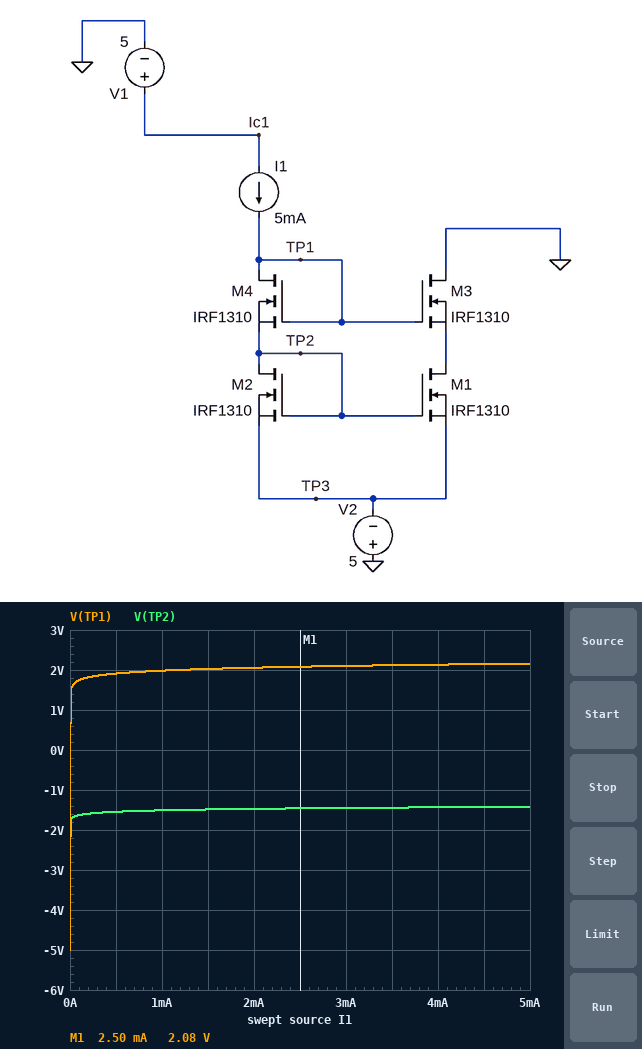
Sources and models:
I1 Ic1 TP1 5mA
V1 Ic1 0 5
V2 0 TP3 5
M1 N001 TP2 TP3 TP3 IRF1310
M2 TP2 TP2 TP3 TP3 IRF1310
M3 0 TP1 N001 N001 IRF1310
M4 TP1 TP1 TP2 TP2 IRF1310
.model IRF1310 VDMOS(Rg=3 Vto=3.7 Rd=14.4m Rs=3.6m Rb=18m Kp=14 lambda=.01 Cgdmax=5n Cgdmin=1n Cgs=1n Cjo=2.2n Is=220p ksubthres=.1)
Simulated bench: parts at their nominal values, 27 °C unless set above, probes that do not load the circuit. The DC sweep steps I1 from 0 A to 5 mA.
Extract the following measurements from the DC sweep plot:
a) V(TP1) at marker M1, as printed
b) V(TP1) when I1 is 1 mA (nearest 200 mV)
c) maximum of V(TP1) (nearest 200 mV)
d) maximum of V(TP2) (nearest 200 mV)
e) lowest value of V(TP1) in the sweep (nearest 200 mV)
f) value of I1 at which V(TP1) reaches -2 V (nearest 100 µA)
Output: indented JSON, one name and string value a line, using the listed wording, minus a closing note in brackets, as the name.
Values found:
{
  "V(TP1) at marker M1, as printed": "2.08 V",
  "V(TP1) when I1 is 1 mA": "2.0 V",
  "maximum of V(TP1)": "2.2 V",
  "maximum of V(TP2)": "-1.4 V",
  "lowest value of V(TP1) in the sweep": "-5.0 V",
  "value of I1 at which V(TP1) reaches -2 V": "0 A"
}
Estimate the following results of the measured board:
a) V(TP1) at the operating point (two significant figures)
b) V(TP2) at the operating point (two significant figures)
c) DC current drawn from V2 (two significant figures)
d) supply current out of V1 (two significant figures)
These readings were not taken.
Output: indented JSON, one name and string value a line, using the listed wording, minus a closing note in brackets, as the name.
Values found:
{
  "V(TP1) at the operating point": "2.2 V",
  "V(TP2) at the operating point": "-1.4 V",
  "DC current drawn from V2": "10 mA",
  "supply current out of V1": "5.0 mA"
}
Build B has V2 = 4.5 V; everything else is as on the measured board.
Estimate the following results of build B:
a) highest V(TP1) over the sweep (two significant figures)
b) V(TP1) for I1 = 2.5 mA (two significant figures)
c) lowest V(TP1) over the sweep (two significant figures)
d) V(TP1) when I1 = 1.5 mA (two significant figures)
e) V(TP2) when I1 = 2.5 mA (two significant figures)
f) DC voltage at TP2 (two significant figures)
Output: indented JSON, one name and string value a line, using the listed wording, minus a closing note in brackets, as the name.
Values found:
{
  "highest V(TP1) over the sweep": "2.7 V",
  "V(TP1) for I1 = 2.5 mA": "2.6 V",
  "lowest V(TP1) over the sweep": "-4.5 V",
  "V(TP1) when I1 = 1.5 mA": "2.5 V",
  "V(TP2) when I1 = 2.5 mA": "-960 mV",
  "DC voltage at TP2": "-920 mV"
}
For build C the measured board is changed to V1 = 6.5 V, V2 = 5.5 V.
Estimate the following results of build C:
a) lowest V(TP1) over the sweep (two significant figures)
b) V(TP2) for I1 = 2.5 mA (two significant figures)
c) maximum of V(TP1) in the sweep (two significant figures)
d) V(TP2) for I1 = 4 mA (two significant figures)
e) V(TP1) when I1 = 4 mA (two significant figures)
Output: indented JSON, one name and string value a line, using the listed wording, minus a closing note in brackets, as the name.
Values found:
{
  "lowest V(TP1) over the sweep": "-5.5 V",
  "V(TP2) for I1 = 2.5 mA": "-2.0 V",
  "maximum of V(TP1) in the sweep": "1.7 V",
  "V(TP2) for I1 = 4 mA": "-1.9 V",
  "V(TP1) when I1 = 4 mA": "1.6 V"
}
